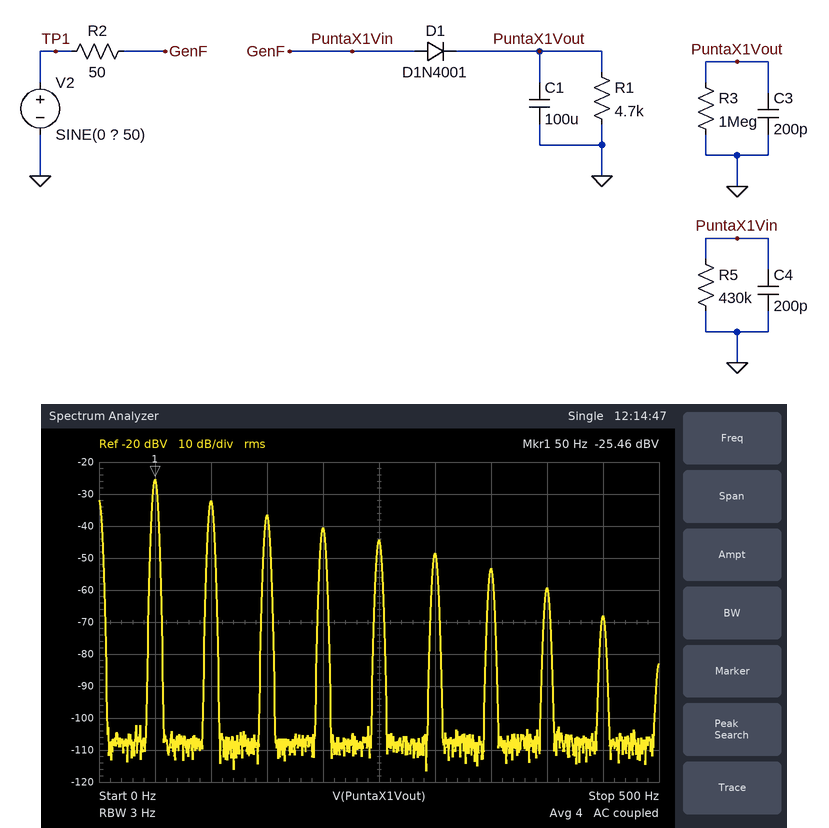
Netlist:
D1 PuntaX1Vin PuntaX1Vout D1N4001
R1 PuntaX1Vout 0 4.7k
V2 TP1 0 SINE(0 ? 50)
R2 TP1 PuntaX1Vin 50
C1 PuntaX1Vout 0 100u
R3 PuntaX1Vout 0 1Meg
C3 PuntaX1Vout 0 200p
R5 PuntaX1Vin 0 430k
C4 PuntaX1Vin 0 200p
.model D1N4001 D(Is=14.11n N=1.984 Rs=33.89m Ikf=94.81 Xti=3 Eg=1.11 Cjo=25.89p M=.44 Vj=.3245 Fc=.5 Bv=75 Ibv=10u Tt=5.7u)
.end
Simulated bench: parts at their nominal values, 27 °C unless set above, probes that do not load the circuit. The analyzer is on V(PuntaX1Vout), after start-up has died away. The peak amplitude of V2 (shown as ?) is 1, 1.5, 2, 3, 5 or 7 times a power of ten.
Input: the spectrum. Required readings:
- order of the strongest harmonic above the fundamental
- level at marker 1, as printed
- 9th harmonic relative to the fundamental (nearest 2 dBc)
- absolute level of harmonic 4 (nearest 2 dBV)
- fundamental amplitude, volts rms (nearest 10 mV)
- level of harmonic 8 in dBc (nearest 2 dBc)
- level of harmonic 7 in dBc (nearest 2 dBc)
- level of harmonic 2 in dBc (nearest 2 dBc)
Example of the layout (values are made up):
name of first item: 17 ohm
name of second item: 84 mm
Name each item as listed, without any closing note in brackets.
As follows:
order of the strongest harmonic above the fundamental: 2
level at marker 1, as printed: -25.46 dBV
9th harmonic relative to the fundamental: -42 dBc
absolute level of harmonic 4: -40 dBV
fundamental amplitude, volts rms: 50 mV
level of harmonic 8 in dBc: -34 dBc
level of harmonic 7 in dBc: -28 dBc
level of harmonic 2 in dBc: -6 dBc
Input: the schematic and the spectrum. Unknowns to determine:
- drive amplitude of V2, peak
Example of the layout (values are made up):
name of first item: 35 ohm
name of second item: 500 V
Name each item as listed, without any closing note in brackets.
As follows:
drive amplitude of V2, peak: 7 V
